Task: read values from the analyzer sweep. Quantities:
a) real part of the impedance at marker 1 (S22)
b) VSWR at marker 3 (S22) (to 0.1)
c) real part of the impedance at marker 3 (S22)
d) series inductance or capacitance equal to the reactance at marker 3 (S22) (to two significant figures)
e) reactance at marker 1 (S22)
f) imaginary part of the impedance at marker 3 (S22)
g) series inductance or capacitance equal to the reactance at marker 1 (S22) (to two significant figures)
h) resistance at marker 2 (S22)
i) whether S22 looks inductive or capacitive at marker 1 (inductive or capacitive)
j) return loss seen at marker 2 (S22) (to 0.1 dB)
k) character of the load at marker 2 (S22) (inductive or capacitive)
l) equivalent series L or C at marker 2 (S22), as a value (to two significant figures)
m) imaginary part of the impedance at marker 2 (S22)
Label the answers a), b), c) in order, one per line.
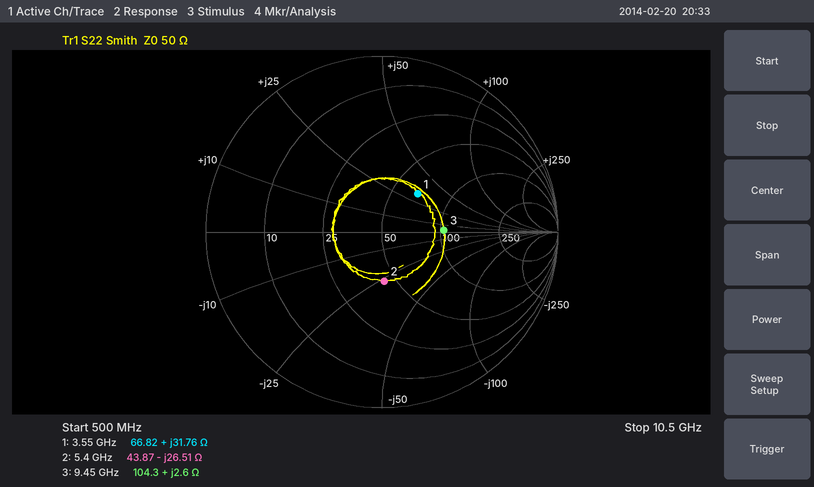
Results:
a) 66.82 Ω
b) 2.1
c) 104.3 Ω
d) 44 pH
e) +31.76 Ω
f) +2.6 Ω
g) 1.4 nH
h) 43.87 Ω
i) inductive
j) 11.1 dB
k) capacitive
l) 1.1 pF
m) -26.51 Ω
